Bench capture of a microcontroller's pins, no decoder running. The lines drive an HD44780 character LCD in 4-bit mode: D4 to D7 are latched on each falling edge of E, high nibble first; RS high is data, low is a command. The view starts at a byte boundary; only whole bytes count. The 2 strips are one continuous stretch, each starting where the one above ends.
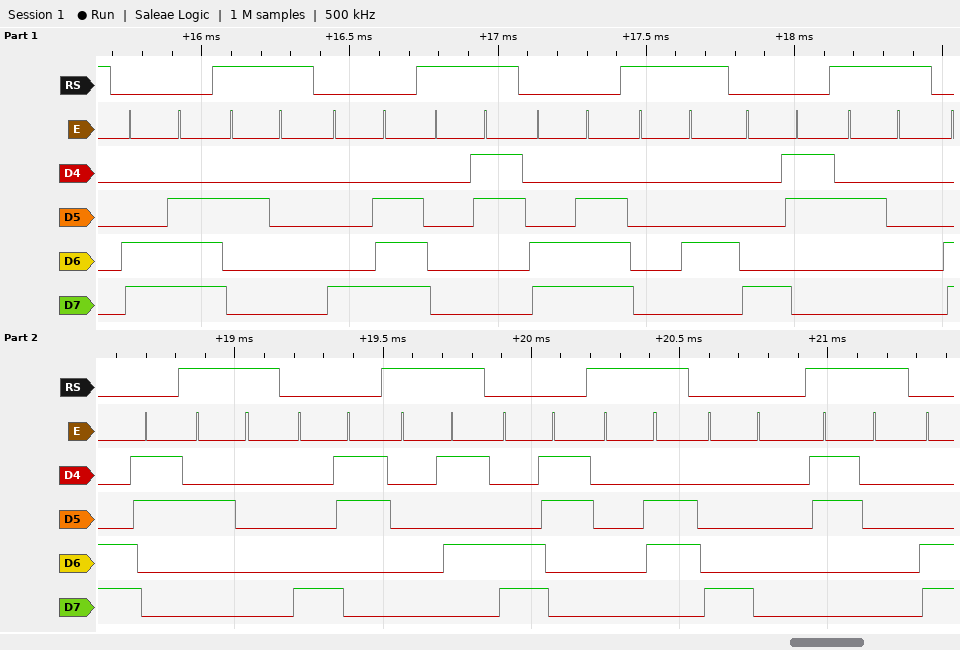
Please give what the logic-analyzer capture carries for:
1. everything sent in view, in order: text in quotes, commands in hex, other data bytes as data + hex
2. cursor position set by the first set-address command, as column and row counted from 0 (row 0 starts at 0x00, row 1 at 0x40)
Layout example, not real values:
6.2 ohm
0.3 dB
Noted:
0xCE " " 0x8E data 03 0xCE data 04 0x83 " " 0xC3 " " 0x83 data 05 0xC3 data 06 0x80 "0"
column 14, row 1
